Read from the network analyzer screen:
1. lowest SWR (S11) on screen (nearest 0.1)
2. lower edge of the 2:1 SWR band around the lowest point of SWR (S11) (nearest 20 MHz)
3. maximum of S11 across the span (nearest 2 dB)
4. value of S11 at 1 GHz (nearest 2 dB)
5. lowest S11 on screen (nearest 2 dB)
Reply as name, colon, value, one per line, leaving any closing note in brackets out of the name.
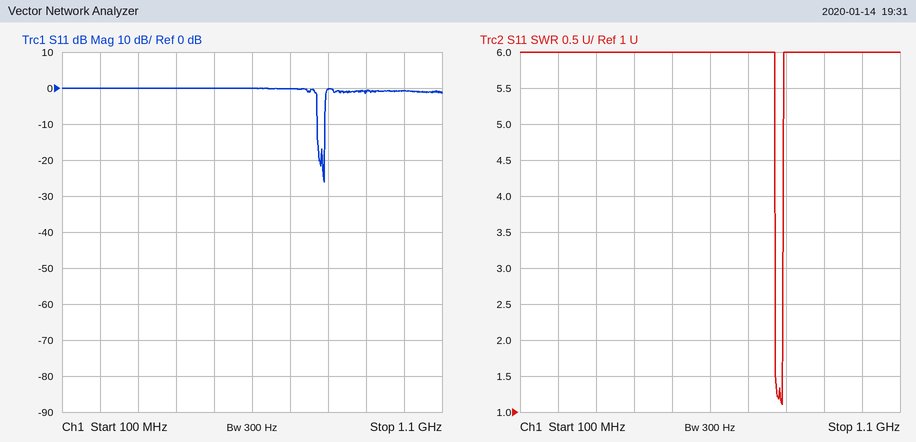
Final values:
lowest SWR (S11) on screen: 1.1
lower edge of the 2:1 SWR band around the lowest point of SWR (S11): 780 MHz
maximum of S11 across the span: 0 dB
value of S11 at 1 GHz: 0 dB
lowest S11 on screen: -26 dB
